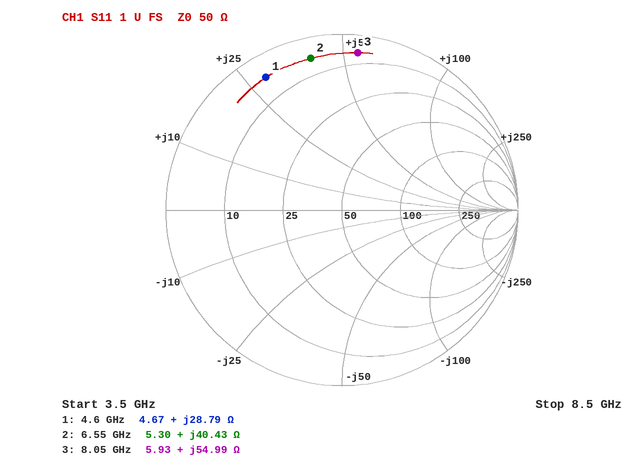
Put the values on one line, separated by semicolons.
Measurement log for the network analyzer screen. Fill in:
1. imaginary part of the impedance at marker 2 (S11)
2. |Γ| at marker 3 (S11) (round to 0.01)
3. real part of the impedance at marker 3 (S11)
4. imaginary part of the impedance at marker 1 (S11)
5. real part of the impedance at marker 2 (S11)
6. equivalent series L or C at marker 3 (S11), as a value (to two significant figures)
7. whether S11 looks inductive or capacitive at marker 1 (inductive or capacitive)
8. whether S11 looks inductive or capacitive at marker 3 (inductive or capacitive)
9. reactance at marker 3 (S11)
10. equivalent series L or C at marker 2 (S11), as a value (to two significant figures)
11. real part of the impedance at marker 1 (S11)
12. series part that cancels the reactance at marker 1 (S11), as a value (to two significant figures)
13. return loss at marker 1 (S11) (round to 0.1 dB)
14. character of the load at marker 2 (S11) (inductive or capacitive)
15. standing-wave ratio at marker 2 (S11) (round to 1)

+40.43 Ω; 0.90; 5.93 Ω; +28.79 Ω; 5.30 Ω; 1.1 nH; inductive; inductive; +54.99 Ω; 980 pH; 4.67 Ω; 1.2 pF; 1.2 dB; inductive; 16
